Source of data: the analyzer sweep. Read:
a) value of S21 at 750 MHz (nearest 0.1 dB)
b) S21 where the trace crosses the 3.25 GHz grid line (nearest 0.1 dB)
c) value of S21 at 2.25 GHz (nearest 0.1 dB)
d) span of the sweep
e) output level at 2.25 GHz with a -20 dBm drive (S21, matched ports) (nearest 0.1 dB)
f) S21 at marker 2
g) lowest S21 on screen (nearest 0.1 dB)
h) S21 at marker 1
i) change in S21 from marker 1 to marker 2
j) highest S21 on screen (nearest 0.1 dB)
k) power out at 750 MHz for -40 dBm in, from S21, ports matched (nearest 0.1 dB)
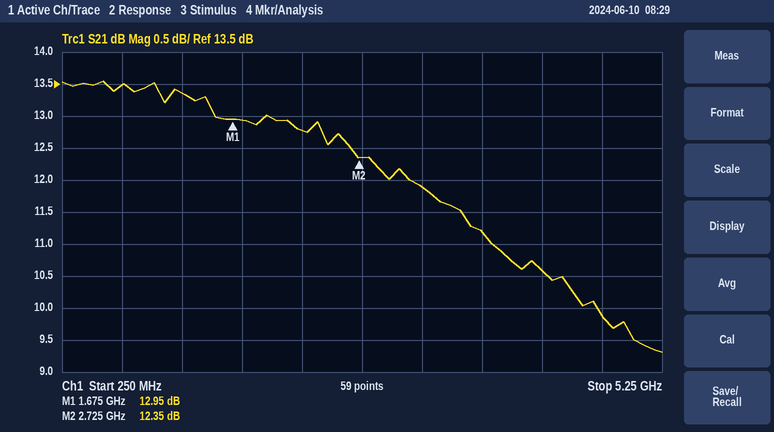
13.5 dB
11.9 dB
12.8 dB
5 GHz
-7.2 dBm
12.35 dB
9.3 dB
12.95 dB
-0.60 dB
13.5 dB
-26.5 dBm
